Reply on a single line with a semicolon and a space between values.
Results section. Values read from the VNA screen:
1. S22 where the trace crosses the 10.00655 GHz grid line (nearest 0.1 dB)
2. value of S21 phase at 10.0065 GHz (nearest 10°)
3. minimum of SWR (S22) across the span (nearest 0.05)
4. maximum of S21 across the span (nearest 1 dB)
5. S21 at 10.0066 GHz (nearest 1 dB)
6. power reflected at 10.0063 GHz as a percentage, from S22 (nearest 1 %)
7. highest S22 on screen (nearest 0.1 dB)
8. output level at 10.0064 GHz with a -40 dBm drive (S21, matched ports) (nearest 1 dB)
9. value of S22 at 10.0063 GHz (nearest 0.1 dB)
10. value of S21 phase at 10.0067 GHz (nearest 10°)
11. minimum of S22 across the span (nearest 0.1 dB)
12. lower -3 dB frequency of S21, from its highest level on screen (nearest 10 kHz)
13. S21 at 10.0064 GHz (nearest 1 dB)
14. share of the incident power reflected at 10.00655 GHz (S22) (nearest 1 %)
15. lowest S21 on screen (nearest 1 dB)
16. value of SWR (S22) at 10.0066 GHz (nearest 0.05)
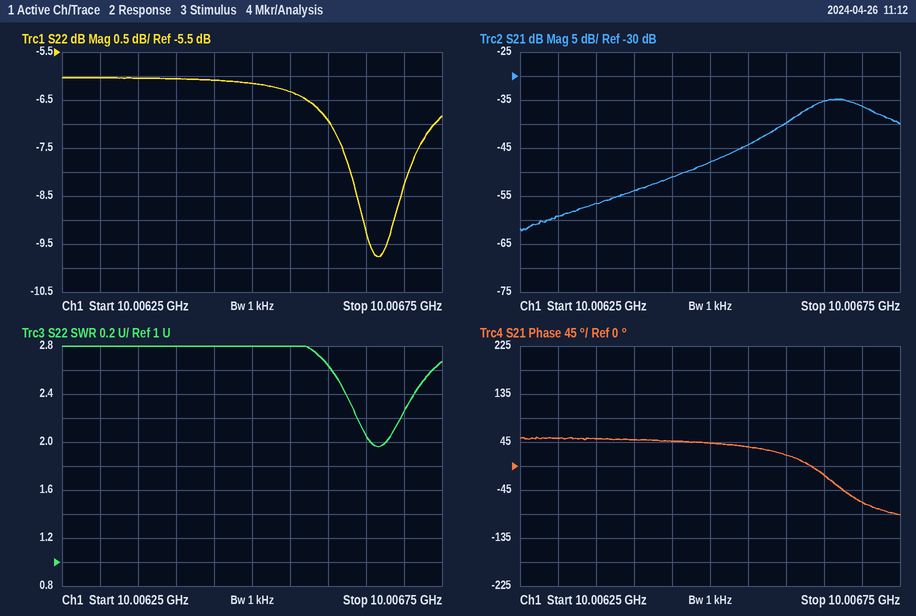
-6.3 dB; 40°; 1.95; -35 dB; -40 dB; 25 %; -6.0 dB; -94 dBm; -6.0 dB; -70°; -9.8 dB; 10.00662 GHz; -54 dB; 23 %; -62 dB; 2.65
